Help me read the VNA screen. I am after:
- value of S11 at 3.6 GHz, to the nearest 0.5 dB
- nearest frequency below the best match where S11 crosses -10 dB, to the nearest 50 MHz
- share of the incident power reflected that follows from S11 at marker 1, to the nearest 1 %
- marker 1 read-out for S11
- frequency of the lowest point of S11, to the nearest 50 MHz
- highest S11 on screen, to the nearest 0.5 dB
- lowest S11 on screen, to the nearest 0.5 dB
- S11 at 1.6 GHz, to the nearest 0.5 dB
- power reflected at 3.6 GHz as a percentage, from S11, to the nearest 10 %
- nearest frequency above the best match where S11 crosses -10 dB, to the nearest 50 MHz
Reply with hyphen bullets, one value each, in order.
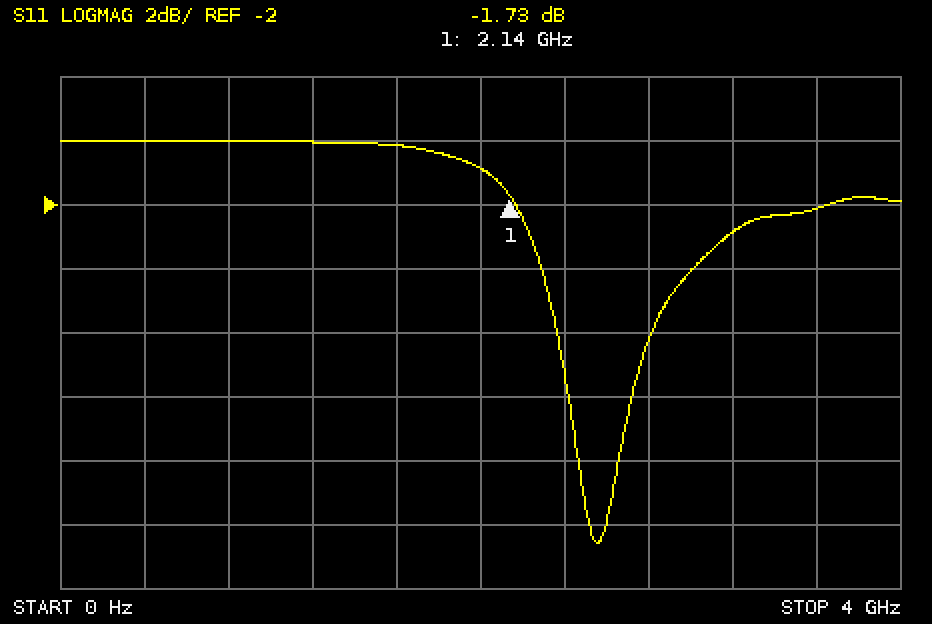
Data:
- -2.0 dB
- 2.45 GHz
- 67 %
- -1.73 dB
- 2.55 GHz
- 0.0 dB
- -12.5 dB
- 0.0 dB
- 60 %
- 2.65 GHz
